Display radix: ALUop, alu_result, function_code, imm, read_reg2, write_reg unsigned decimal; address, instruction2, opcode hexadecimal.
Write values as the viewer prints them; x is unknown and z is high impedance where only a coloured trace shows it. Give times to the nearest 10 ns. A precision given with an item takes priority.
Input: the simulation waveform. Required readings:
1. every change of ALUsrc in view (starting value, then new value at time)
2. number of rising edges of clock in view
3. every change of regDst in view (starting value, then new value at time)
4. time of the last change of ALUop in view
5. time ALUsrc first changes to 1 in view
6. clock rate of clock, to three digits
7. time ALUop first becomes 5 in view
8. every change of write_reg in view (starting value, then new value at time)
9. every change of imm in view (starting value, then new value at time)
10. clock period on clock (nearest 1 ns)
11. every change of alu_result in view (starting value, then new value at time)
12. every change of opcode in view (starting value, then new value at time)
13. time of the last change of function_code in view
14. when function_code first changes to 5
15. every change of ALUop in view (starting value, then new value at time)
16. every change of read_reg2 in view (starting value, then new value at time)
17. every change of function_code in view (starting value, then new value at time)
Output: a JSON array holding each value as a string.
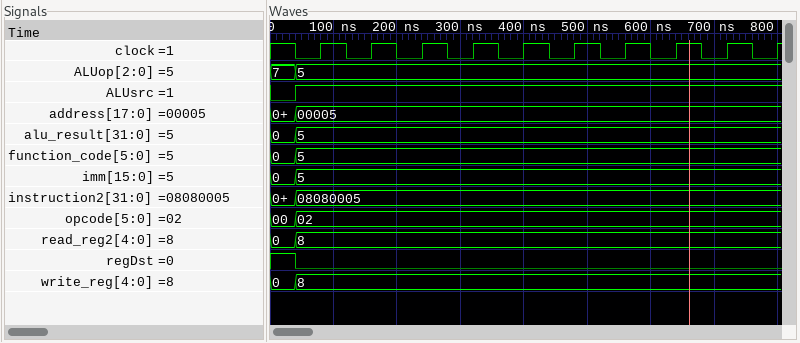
["0, 1 at 40 ns", "10", "1, 0 at 40 ns", "40 ns", "40 ns", "12.5 MHz", "40 ns", "0, 8 at 40 ns", "0, 5 at 40 ns", "80 ns", "0, 5 at 40 ns", "00, 02 at 40 ns", "40 ns", "40 ns", "7, 5 at 40 ns", "0, 8 at 40 ns", "0, 5 at 40 ns"]
